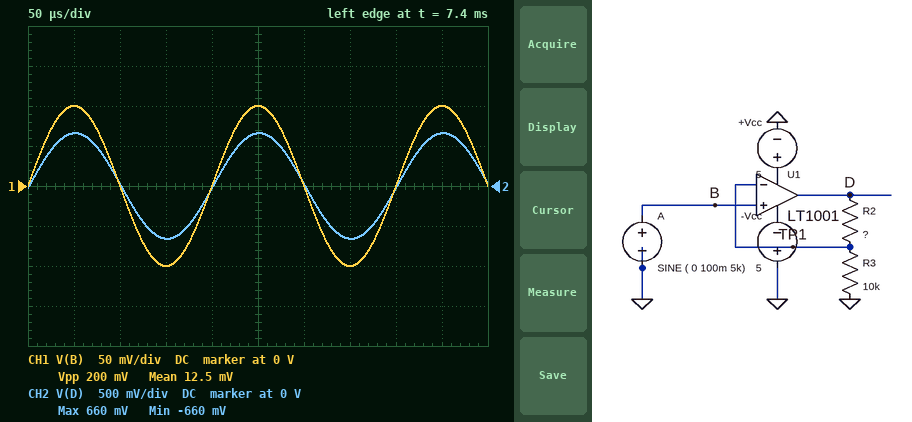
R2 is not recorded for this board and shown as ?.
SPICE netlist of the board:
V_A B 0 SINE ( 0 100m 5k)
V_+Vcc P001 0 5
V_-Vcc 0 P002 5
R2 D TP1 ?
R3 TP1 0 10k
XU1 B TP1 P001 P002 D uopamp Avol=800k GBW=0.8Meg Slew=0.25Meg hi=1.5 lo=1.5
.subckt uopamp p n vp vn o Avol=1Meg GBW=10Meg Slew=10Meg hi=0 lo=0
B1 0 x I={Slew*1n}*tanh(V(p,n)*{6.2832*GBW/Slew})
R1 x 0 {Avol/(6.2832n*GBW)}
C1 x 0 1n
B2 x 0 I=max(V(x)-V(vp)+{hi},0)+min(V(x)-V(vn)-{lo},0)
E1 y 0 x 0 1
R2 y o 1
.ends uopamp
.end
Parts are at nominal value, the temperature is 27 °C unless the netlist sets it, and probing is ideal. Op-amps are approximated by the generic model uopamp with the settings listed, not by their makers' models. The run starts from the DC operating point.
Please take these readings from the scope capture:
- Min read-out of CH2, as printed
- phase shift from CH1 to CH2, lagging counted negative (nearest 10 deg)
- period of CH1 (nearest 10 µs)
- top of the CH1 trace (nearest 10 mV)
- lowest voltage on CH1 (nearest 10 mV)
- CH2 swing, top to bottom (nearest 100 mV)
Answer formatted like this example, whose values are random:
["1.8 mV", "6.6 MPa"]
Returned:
["-660 mV", "0 deg", "200 µs", "100 mV", "-100 mV", "1.3 V"]
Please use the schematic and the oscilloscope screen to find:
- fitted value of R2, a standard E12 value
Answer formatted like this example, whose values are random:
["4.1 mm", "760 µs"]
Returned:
["56 kΩ"]
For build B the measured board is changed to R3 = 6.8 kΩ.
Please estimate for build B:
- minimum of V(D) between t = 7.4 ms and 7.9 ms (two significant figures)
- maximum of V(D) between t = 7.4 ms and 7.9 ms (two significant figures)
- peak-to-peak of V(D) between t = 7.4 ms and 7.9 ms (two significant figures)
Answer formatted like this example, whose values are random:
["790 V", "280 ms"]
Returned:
["-920 mV", "920 mV", "1.8 V"]
